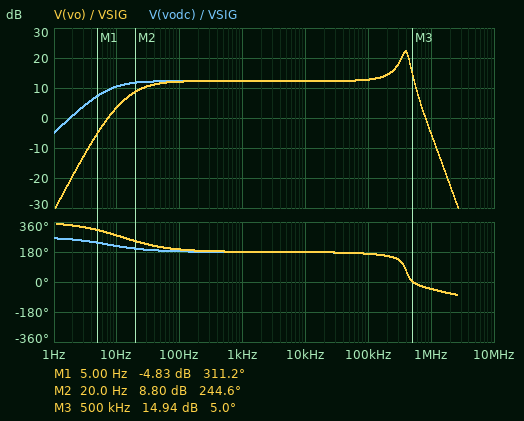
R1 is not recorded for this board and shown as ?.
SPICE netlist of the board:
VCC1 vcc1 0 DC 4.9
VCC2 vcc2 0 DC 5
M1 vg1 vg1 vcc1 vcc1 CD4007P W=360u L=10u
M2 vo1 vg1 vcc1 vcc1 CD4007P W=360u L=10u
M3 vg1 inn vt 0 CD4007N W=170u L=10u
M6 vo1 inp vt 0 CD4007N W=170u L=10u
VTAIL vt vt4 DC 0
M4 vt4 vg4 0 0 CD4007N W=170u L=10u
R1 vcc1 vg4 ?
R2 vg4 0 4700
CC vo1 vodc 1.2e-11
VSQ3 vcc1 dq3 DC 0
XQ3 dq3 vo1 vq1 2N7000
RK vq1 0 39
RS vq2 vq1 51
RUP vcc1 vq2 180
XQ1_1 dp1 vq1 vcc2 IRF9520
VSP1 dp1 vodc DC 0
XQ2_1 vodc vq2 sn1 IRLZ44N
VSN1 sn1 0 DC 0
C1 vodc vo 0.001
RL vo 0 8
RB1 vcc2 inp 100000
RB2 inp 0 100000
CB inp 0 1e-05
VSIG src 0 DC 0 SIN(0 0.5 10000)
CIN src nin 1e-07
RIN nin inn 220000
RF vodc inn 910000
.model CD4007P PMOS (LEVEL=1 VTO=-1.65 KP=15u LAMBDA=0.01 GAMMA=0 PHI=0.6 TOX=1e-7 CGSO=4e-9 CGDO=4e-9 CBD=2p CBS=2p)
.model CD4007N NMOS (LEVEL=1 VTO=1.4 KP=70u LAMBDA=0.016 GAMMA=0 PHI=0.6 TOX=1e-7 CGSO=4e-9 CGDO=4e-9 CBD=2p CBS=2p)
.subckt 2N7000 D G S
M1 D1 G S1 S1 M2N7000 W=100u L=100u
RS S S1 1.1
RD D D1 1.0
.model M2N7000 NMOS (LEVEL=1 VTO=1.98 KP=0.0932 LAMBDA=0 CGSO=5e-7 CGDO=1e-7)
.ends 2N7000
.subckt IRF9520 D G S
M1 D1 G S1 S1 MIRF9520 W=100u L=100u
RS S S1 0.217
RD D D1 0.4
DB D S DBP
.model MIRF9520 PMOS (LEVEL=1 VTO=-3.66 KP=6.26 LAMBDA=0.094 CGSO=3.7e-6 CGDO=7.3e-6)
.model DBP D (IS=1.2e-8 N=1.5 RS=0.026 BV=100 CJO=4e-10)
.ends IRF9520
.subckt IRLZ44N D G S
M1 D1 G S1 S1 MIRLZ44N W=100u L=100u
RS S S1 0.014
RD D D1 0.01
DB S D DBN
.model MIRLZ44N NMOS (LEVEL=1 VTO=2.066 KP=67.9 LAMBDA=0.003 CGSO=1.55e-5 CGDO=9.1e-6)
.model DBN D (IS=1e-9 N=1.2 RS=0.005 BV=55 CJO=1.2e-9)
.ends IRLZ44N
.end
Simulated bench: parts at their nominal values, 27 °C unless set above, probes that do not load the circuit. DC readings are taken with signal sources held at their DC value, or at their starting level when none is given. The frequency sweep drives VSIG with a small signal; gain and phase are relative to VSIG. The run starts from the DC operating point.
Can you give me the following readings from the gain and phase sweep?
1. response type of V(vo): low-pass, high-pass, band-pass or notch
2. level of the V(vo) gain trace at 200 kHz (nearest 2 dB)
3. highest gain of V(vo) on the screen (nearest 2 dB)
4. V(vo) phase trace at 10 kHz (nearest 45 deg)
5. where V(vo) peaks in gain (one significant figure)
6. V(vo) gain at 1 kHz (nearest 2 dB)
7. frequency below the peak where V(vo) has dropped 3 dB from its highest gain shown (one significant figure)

band-pass
14 dB
22 dB
180 deg
400 kHz
12 dB
300 kHz
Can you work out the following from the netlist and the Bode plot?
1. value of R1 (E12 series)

8.2 kΩ
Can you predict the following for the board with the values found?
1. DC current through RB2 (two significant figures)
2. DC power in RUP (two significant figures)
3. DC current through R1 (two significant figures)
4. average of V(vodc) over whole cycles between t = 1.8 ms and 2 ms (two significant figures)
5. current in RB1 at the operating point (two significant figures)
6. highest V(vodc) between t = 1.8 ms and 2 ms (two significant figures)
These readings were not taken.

25 µA
44 mW
380 µA
2.5 V
25 µA
4.6 V
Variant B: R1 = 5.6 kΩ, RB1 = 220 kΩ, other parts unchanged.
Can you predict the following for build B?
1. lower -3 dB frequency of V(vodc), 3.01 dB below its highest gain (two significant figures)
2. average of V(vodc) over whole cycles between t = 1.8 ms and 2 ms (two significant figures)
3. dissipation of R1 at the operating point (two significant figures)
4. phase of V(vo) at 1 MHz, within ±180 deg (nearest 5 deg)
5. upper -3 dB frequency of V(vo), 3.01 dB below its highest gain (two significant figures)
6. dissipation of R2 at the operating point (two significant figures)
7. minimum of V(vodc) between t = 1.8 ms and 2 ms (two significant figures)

160 kHz
1.6 V
1.3 mW
-60 deg
310 kHz
1.1 mW
10 mV
